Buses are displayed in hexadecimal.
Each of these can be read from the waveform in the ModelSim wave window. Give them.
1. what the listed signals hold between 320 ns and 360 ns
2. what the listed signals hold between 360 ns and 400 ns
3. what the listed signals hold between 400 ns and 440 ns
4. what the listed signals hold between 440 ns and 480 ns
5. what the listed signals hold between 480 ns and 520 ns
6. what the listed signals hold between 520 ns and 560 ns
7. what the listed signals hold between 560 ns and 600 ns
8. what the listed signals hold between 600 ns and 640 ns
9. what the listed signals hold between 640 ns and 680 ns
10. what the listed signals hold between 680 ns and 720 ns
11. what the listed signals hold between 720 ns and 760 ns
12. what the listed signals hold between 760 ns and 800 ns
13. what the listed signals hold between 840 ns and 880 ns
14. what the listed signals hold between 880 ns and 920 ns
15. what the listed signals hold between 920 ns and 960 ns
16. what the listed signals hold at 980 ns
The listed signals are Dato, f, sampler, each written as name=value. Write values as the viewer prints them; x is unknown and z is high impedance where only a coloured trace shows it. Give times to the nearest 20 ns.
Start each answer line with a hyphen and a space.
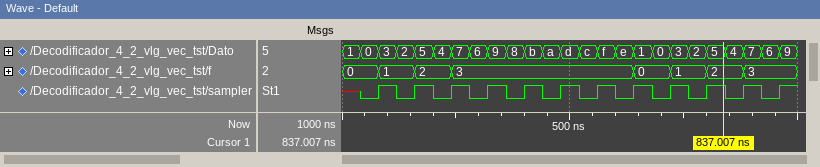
- Dato=9, f=3, sampler=1
- Dato=8, f=3, sampler=0
- Dato=b, f=3, sampler=1
- Dato=a, f=3, sampler=0
- Dato=d, f=3, sampler=1
- Dato=c, f=3, sampler=0
- Dato=f, f=3, sampler=1
- Dato=e, f=3, sampler=0
- Dato=1, f=0, sampler=1
- Dato=0, f=0, sampler=0
- Dato=3, f=1, sampler=1
- Dato=2, f=1, sampler=0
- Dato=4, f=2, sampler=0
- Dato=7, f=3, sampler=1
- Dato=6, f=3, sampler=0
- Dato=9, f=3, sampler=1
